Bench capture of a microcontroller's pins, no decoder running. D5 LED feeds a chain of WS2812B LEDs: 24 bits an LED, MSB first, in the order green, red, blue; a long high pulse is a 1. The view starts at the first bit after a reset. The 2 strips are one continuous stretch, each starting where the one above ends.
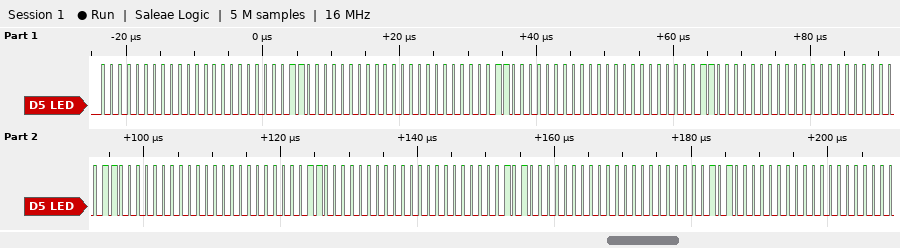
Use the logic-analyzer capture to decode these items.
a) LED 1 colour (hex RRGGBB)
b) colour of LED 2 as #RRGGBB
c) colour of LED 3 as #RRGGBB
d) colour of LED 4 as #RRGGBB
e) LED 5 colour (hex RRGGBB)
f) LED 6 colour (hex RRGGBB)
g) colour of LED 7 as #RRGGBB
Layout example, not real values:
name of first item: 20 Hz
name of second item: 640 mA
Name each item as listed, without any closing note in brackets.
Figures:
LED 1 colour: #000003
colour of LED 2 as #RRGGBB: #000003
colour of LED 3 as #RRGGBB: #000003
colour of LED 4 as #RRGGBB: #000003
LED 5 colour: #000003
LED 6 colour: #000005
colour of LED 7 as #RRGGBB: #000005
